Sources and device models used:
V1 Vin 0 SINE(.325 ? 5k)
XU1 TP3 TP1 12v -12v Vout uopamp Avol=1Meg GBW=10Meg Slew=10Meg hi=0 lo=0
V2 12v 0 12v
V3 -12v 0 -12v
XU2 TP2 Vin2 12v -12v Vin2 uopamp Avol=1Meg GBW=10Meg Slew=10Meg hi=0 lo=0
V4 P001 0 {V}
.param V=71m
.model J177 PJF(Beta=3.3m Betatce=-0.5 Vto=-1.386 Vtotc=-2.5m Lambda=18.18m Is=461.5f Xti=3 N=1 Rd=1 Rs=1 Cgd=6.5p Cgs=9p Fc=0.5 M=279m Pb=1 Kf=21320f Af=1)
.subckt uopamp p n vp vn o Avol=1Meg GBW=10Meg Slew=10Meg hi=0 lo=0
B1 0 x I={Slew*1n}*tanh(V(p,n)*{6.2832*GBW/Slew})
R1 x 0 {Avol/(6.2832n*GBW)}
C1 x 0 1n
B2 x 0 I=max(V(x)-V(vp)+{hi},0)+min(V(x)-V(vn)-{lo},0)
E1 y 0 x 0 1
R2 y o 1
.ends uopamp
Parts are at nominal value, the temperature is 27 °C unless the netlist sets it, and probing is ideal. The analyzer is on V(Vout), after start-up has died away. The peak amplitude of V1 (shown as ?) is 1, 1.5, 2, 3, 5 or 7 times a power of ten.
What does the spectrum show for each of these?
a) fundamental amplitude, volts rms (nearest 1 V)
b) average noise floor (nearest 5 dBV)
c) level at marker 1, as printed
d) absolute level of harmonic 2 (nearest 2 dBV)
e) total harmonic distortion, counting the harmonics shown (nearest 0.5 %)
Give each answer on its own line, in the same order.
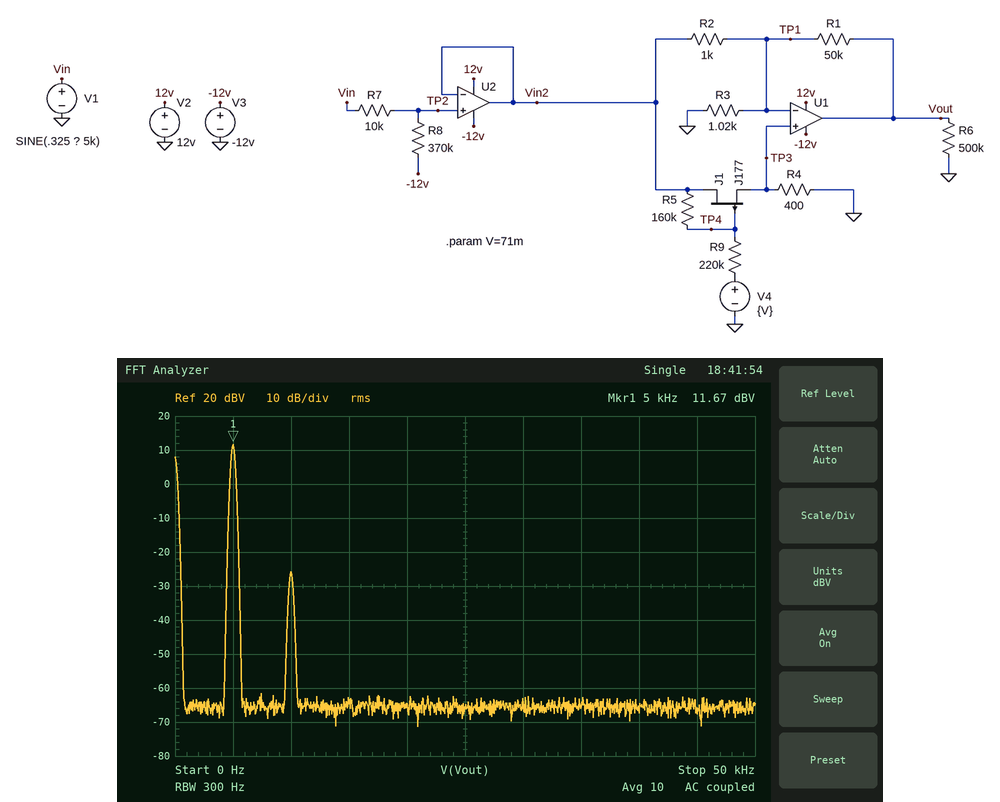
4 V
-65 dBV
11.67 dBV
-26 dBV
1.5 %
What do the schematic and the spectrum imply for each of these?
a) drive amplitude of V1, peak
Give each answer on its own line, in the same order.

200 mV
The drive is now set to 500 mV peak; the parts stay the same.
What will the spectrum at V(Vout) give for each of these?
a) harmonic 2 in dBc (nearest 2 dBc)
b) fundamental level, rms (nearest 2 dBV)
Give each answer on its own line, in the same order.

-58 dBc
20 dBV
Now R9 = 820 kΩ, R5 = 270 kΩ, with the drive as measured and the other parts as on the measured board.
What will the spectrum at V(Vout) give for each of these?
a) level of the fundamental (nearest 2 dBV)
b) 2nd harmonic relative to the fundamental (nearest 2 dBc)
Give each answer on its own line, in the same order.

12 dBV
-44 dBc
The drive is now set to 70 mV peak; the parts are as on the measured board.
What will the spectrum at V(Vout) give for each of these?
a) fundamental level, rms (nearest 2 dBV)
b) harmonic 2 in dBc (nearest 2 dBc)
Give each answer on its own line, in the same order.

2 dBV
-46 dBc
